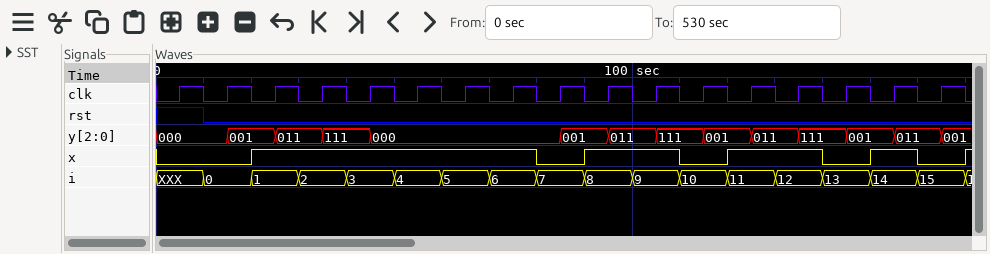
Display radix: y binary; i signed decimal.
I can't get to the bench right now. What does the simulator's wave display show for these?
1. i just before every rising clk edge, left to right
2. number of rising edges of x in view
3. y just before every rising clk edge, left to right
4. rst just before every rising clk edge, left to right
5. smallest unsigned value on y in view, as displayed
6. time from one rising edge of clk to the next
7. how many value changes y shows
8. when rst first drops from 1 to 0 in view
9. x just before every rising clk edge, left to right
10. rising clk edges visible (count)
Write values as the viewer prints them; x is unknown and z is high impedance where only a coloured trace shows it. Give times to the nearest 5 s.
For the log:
XXX, 0, 1, 2, 3, 4, 5, 6, 7, 8, 9, 10, 11, 12, 13, 14, 15
5
000, 000, 001, 011, 111, 000, 000, 000, 000, 001, 011, 111, 001, 011, 111, 001, 011
1 0 0 0 0 0 0 0 0 0 0 0 0 0 0 0 0
000
10 s
13
10 s
0 0 1 1 1 1 1 1 0 1 1 0 1 1 0 1 0
17
